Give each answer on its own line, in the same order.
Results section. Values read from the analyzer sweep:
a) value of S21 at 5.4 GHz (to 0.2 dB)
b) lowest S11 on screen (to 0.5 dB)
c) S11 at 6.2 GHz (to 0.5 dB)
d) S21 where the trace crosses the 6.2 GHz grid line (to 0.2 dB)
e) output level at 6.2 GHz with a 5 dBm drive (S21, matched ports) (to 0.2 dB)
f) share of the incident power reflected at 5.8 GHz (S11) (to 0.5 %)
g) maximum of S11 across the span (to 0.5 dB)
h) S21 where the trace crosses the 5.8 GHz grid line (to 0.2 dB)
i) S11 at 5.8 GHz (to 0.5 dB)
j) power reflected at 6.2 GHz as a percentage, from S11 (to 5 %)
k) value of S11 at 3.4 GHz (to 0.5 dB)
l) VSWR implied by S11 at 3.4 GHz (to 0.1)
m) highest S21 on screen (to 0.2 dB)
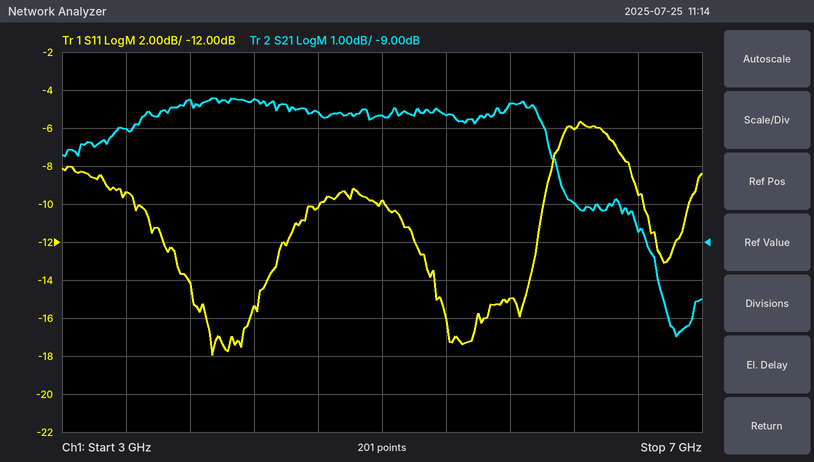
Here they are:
-5.6 dB
-18.0 dB
-6.0 dB
-8.0 dB
-3.0 dBm
3.0 %
-5.5 dB
-5.4 dB
-15.0 dB
25 %
-9.5 dB
2.0
-5.2 dB
